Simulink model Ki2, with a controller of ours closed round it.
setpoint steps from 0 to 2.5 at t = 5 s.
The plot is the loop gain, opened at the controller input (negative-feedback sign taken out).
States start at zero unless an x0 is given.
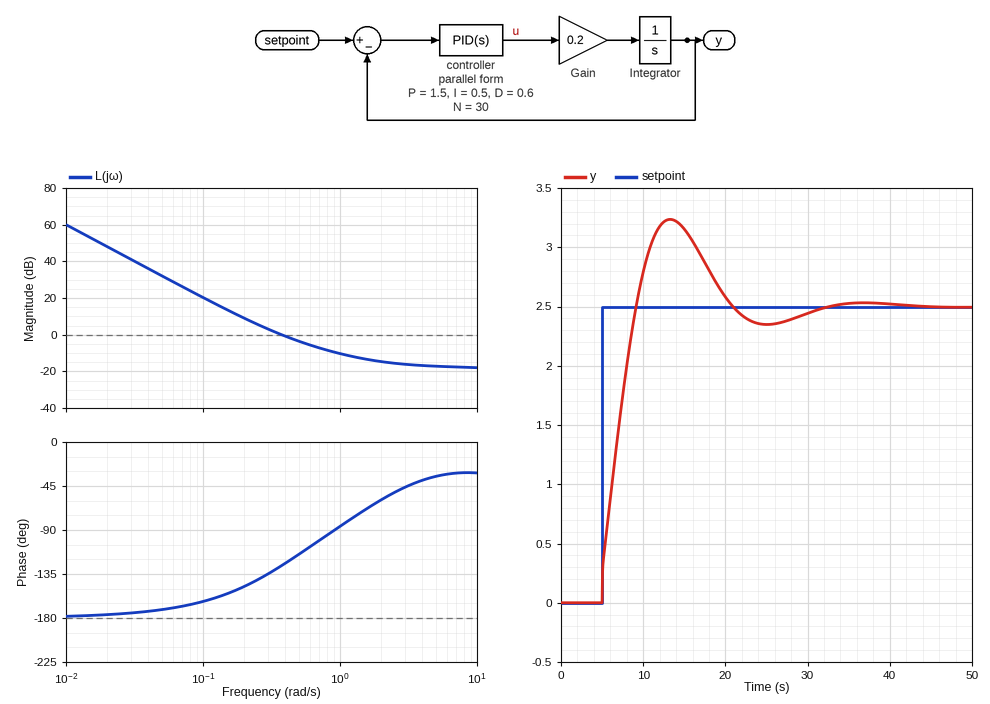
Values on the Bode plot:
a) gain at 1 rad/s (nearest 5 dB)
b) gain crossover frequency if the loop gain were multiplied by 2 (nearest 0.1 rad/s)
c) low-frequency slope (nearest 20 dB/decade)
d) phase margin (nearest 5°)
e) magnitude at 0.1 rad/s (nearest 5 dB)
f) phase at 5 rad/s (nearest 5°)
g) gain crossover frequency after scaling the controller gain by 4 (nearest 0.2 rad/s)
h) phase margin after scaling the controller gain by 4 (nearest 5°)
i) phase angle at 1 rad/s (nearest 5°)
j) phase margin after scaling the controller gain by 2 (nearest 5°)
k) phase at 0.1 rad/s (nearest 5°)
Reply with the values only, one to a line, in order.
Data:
-10 dB
0.6 rad/s
-40 dB/decade
55°
20 dB
-35°
1.2 rad/s
105°
-85°
75°
-165°
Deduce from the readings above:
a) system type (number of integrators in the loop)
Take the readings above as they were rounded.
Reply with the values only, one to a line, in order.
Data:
2
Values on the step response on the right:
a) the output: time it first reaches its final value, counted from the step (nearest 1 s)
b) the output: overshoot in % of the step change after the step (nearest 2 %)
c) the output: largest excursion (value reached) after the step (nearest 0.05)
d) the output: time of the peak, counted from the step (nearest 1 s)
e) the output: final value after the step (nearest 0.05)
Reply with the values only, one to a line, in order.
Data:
4 s
30 %
3.25
8 s
2.50
